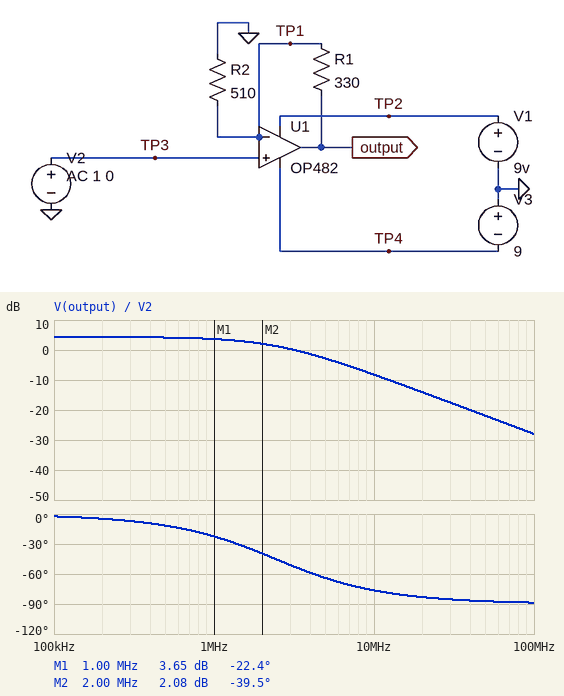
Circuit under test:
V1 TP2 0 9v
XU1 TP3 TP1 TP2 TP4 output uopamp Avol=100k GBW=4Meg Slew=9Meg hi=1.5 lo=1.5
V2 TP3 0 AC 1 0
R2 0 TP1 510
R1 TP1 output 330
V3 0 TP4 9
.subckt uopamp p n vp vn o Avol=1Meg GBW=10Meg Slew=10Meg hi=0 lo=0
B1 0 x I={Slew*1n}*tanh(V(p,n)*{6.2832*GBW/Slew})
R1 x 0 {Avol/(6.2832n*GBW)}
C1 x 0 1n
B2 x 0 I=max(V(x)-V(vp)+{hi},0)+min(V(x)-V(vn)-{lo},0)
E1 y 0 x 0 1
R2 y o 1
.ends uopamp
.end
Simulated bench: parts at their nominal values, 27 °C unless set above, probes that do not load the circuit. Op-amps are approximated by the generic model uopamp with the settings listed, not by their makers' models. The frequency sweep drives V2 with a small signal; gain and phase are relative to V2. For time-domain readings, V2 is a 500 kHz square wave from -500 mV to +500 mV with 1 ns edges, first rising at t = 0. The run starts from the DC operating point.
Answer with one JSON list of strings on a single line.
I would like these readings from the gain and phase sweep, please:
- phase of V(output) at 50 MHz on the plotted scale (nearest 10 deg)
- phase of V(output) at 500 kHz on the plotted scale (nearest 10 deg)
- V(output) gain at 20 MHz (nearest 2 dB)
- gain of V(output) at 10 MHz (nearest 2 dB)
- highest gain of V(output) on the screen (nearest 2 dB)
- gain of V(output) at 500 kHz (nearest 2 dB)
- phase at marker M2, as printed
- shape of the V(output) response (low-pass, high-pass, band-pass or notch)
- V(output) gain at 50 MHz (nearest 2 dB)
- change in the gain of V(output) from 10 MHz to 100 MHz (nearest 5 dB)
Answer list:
["-90 deg", "-10 deg", "-14 dB", "-8 dB", "4 dB", "4 dB", "-39.5 deg", "low-pass", "-22 dB", "-20 dB"]
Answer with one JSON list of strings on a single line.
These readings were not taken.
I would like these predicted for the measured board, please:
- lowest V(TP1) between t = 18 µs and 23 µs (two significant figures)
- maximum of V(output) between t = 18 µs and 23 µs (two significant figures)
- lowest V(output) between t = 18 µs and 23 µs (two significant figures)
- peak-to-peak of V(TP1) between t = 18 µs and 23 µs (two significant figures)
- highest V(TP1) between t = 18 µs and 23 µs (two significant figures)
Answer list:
["-500 mV", "820 mV", "-820 mV", "1.0 V", "500 mV"]
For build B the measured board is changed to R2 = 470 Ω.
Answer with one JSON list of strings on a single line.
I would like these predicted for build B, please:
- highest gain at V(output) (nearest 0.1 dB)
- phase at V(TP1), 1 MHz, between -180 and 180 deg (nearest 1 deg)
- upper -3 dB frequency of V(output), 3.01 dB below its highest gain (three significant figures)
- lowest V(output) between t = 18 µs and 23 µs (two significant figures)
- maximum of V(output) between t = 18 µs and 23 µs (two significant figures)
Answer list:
["4.6 dB", "-23 deg", "2.35 MHz", "-850 mV", "850 mV"]
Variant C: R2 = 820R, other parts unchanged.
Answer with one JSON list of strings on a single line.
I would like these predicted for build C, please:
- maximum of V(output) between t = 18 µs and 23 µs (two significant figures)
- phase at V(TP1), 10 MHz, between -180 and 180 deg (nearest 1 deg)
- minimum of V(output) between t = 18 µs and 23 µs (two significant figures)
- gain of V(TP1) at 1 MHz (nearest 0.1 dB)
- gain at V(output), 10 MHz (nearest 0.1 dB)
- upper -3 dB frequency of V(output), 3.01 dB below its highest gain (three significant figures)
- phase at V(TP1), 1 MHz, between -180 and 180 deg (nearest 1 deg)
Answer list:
["700 mV", "-74 deg", "-700 mV", "-0.5 dB", "-8.3 dB", "2.85 MHz", "-19 deg"]
